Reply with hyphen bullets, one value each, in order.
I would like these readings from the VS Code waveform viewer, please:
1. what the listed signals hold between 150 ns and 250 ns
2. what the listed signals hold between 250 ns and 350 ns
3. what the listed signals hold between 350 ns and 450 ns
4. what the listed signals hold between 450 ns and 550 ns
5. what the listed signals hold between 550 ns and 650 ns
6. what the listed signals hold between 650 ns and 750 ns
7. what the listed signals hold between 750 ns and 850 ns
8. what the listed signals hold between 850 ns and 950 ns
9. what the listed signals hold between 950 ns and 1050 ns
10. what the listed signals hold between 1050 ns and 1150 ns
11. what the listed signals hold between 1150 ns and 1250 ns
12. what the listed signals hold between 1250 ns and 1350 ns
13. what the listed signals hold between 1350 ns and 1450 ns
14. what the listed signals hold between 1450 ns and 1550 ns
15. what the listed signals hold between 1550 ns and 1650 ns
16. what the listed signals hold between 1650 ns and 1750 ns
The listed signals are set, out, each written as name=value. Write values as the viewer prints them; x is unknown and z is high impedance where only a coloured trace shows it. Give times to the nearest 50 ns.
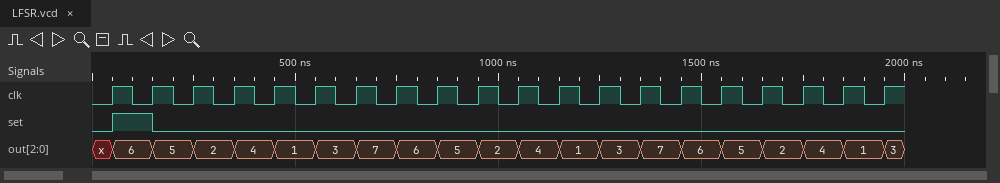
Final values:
- set=0, out=5
- set=0, out=2
- set=0, out=4
- set=0, out=1
- set=0, out=3
- set=0, out=7
- set=0, out=6
- set=0, out=5
- set=0, out=2
- set=0, out=4
- set=0, out=1
- set=0, out=3
- set=0, out=7
- set=0, out=6
- set=0, out=5
- set=0, out=2
